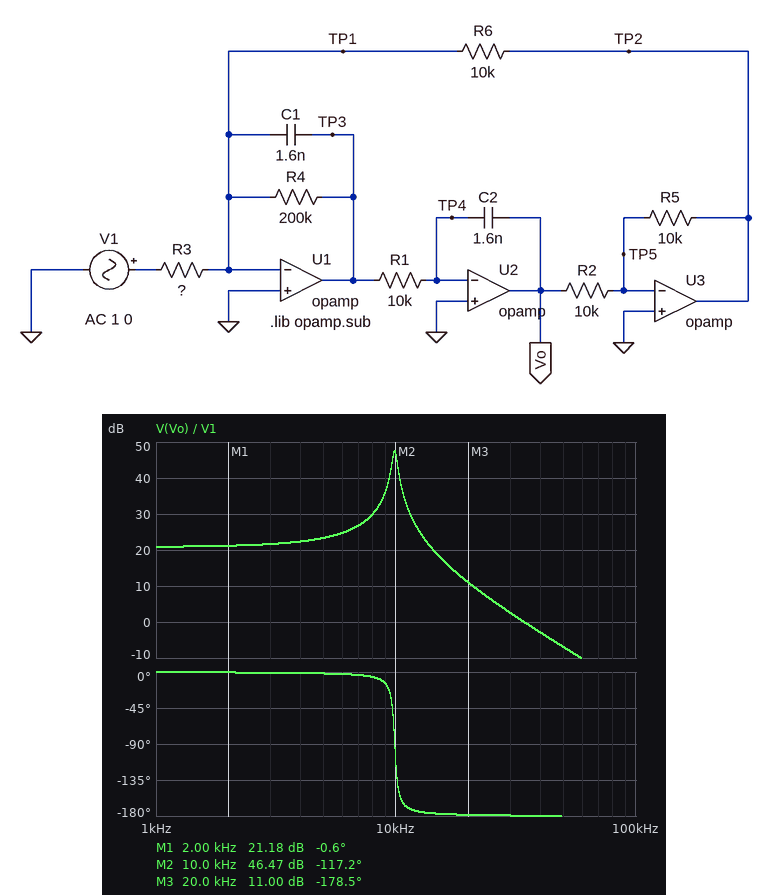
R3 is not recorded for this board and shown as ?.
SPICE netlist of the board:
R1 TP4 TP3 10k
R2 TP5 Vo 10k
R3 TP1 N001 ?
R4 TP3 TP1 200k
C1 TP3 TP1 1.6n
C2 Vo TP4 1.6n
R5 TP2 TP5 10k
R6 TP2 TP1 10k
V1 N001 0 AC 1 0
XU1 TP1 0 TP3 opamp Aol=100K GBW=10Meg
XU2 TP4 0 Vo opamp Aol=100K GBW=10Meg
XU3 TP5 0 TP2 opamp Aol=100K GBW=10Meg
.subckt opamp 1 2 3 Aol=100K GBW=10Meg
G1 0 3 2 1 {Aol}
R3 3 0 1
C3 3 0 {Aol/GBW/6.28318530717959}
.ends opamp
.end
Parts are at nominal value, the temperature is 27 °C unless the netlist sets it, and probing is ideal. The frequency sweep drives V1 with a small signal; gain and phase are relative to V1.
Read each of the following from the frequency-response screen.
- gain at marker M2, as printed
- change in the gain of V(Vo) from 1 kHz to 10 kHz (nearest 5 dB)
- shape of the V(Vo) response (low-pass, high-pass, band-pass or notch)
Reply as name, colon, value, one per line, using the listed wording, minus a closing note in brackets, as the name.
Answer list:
gain at marker M2, as printed: 46.47 dB
change in the gain of V(Vo) from 1 kHz to 10 kHz: 25 dB
shape of the V(Vo) response: low-pass
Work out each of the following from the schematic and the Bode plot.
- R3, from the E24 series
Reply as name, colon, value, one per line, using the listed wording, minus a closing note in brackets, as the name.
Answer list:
R3, from the E24 series: 910 Ω
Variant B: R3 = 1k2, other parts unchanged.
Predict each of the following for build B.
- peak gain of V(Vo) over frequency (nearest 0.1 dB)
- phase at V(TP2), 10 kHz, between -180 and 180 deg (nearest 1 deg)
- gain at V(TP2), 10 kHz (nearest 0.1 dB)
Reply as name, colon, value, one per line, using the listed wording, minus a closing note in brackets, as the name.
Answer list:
peak gain of V(Vo) over frequency: 45.2 dB
phase at V(TP2), 10 kHz, between -180 and 180 deg: 65 deg
gain at V(TP2), 10 kHz: 44.3 dB
